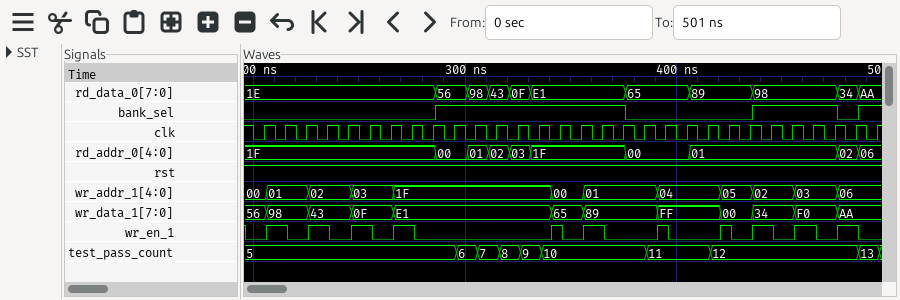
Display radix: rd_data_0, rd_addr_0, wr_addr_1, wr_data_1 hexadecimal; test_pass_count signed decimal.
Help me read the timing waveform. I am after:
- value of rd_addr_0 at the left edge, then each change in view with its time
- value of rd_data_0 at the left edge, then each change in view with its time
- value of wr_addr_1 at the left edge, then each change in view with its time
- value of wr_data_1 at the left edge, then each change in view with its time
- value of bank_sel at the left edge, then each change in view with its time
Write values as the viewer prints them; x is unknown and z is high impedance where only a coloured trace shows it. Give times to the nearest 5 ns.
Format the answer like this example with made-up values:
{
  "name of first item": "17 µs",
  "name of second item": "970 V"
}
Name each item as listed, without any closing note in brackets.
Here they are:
{
  "value of rd_addr_0 at the left edge, then each change in view with its time": "1F, 00 at 285 ns, 01 at 300 ns, 02 at 310 ns, 03 at 320 ns, 1F at 330 ns, 00 at 375 ns, 01 at 405 ns, 02 at 475 ns, 06 at 485 ns",
  "value of rd_data_0 at the left edge, then each change in view with its time": "1E, 56 at 285 ns, 98 at 300 ns, 43 at 310 ns, 0F at 320 ns, E1 at 330 ns, 65 at 375 ns, 89 at 405 ns, 98 at 435 ns, 34 at 475 ns, AA at 485 ns",
  "value of wr_addr_1 at the left edge, then each change in view with its time": "00, 01 at 205 ns, 02 at 225 ns, 03 at 245 ns, 1F at 265 ns, 00 at 340 ns, 01 at 355 ns, 04 at 390 ns, 05 at 420 ns, 02 at 435 ns, 03 at 455 ns, 06 at 475 ns",
  "value of wr_data_1 at the left edge, then each change in view with its time": "56, 98 at 205 ns, 43 at 225 ns, 0F at 245 ns, E1 at 265 ns, 65 at 340 ns, 89 at 355 ns, FF at 390 ns, 00 at 420 ns, 34 at 435 ns, F0 at 455 ns, AA at 475 ns",
  "value of bank_sel at the left edge, then each change in view with its time": "0, 1 at 285 ns, 0 at 375 ns, 1 at 435 ns, 0 at 475 ns, 1 at 485 ns"
}
